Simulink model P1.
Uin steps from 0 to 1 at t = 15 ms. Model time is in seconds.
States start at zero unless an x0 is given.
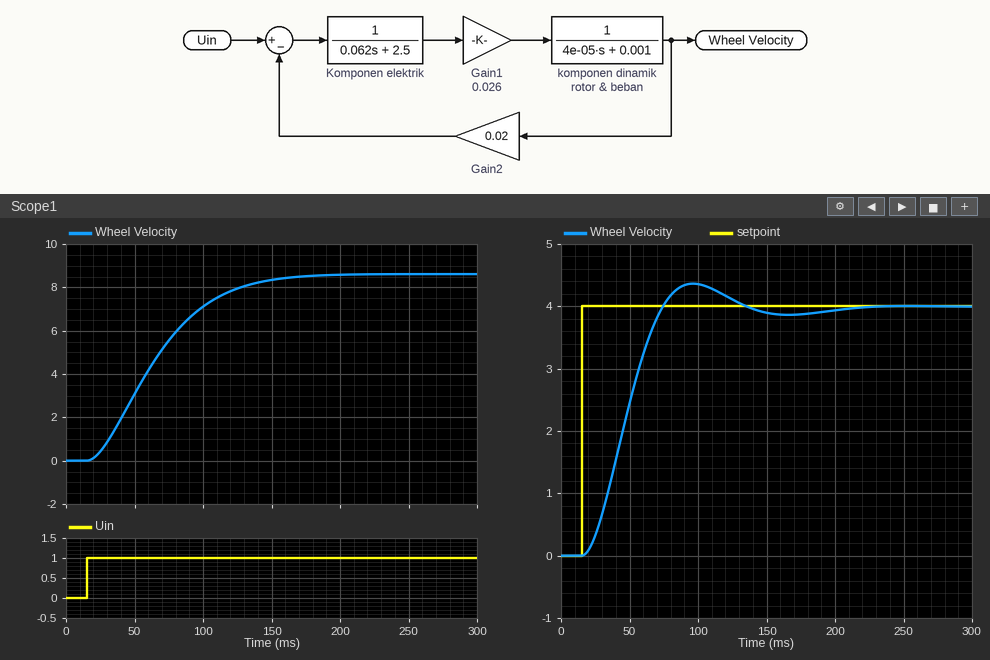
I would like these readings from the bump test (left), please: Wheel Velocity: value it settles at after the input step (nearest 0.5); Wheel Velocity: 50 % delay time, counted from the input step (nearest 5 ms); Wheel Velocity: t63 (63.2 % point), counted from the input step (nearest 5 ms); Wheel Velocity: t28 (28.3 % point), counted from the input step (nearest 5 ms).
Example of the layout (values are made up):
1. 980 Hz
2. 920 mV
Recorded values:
1. 8.5
2. 45 ms
3. 60 ms
4. 30 ms
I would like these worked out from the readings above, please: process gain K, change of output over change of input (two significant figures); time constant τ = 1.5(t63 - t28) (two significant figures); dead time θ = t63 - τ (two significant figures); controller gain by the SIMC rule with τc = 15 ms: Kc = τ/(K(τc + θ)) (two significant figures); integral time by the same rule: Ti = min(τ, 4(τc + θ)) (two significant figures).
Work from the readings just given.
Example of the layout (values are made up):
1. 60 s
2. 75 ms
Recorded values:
1. 8.5
2. 45 ms
3. 15 ms
4. 0.18
5. 45 ms
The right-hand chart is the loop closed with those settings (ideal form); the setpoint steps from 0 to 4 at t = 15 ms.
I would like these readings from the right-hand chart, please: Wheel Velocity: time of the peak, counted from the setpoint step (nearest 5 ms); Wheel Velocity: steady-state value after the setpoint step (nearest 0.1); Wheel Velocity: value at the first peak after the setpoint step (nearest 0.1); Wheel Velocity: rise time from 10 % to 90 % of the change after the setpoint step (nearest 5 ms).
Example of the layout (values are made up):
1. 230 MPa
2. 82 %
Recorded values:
1. 80 ms
2. 4.0
3. 4.4
4. 40 ms
